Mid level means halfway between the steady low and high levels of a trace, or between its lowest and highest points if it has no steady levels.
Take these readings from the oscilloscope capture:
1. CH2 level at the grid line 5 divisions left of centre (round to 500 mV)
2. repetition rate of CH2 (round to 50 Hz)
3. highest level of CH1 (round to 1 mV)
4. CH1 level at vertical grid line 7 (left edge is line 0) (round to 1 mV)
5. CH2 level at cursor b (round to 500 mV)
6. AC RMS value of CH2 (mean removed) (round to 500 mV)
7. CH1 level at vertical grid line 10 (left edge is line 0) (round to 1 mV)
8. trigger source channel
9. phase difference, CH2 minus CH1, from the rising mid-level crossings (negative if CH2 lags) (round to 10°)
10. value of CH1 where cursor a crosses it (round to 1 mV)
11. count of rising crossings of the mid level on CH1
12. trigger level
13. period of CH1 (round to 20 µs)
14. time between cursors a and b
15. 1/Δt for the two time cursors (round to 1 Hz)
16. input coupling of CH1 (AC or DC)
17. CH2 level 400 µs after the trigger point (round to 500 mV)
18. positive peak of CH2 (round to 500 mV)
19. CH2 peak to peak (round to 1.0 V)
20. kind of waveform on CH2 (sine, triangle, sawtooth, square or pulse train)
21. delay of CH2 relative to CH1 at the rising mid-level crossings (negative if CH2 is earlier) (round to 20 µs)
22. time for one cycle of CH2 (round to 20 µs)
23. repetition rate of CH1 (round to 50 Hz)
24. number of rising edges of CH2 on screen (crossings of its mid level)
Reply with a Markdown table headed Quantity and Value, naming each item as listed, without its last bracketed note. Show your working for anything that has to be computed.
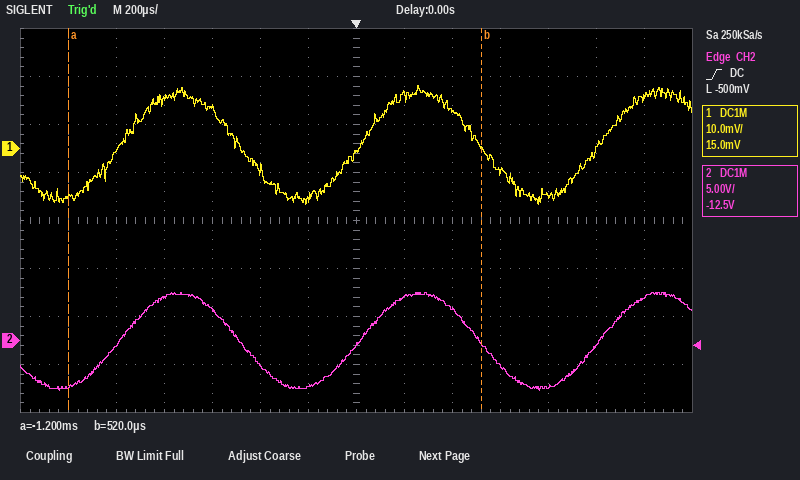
| Quantity | Value |
|---|---|
| CH2 level at the grid line 5 divisions left of centre | -500 mV |
| repetition rate of CH2 | 1 / 1.00 ms ≈ 1.00 kHz |
| highest level of CH1 | 13 mV |
| CH1 level at vertical grid line 7 (left edge is line 0) | -1 mV |
| CH2 level at cursor b | 0.0 V |
| AC RMS value of CH2 (mean removed) | 10.0 V / (2√2) ≈ 3.5 V |
| CH1 level at vertical grid line 10 (left edge is line 0) | -5 mV |
| trigger source channel | CH2 |
| phase difference, CH2 minus CH1, from the rising mid-level crossings (negative if CH2 lags) | −360° × (0 µs) / 1.00 ms ≈ 0° |
| value of CH1 where cursor a crosses it | -10 mV |
| count of rising crossings of the mid level on CH1 | 3 |
| trigger level | -500 mV |
| period of CH1 | 1.00 ms |
| time between cursors a and b | 520 µs − (-1.2 ms) = 1.72 ms |
| 1/Δt for the two time cursors | 1 / 1.72 ms ≈ 581 Hz |
| input coupling of CH1 | DC |
| CH2 level 400 µs after the trigger point | 3.5 V |
| positive peak of CH2 | 5.0 V |
| CH2 peak to peak | 10.0 V |
| kind of waveform on CH2 | sine |
| delay of CH2 relative to CH1 at the rising mid-level crossings (negative if CH2 is earlier) | 0 µs |
| time for one cycle of CH2 | 1.00 ms |
| repetition rate of CH1 | 1 / 1.00 ms ≈ 1.00 kHz |
| number of rising edges of CH2 on screen | 3 |
